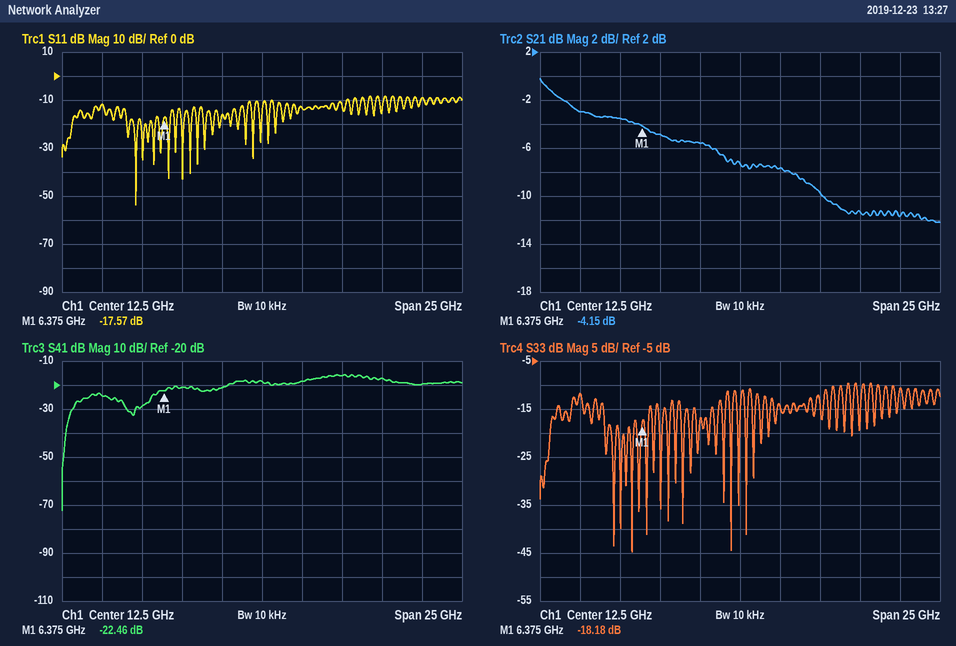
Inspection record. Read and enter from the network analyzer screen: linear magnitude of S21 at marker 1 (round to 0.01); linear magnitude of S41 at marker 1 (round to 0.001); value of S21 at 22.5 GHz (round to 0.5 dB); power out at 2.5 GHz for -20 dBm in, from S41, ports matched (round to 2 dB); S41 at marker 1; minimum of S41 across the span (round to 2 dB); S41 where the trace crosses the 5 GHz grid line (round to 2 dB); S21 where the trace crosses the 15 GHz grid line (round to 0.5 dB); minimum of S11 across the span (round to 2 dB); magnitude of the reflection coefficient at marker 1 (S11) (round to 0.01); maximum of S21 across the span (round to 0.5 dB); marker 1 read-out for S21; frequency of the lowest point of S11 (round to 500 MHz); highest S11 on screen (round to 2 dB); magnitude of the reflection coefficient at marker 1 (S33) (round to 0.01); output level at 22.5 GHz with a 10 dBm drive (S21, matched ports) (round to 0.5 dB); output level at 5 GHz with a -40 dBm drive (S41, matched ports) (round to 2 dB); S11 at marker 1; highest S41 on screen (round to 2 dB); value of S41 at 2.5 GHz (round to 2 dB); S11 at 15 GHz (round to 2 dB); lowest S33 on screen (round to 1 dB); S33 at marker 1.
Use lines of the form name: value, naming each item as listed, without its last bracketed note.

linear magnitude of S21 at marker 1: 0.62
linear magnitude of S41 at marker 1: 0.075
value of S21 at 22.5 GHz: -11.5 dB
power out at 2.5 GHz for -20 dBm in, from S41, ports matched: -44 dBm
S41 at marker 1: -22.46 dB
minimum of S41 across the span: -72 dB
S41 where the trace crosses the 5 GHz grid line: -28 dB
S21 where the trace crosses the 15 GHz grid line: -7.5 dB
minimum of S11 across the span: -54 dB
magnitude of the reflection coefficient at marker 1 (S11): 0.13
maximum of S21 across the span: 0.0 dB
marker 1 read-out for S21: -4.15 dB
frequency of the lowest point of S11: 4.5 GHz
highest S11 on screen: -8 dB
magnitude of the reflection coefficient at marker 1 (S33): 0.12
output level at 22.5 GHz with a 10 dBm drive (S21, matched ports): -1.5 dBm
output level at 5 GHz with a -40 dBm drive (S41, matched ports): -68 dBm
S11 at marker 1: -17.57 dB
highest S41 on screen: -16 dB
value of S41 at 2.5 GHz: -24 dB
S11 at 15 GHz: -14 dB
lowest S33 on screen: -45 dB
S33 at marker 1: -18.18 dB
